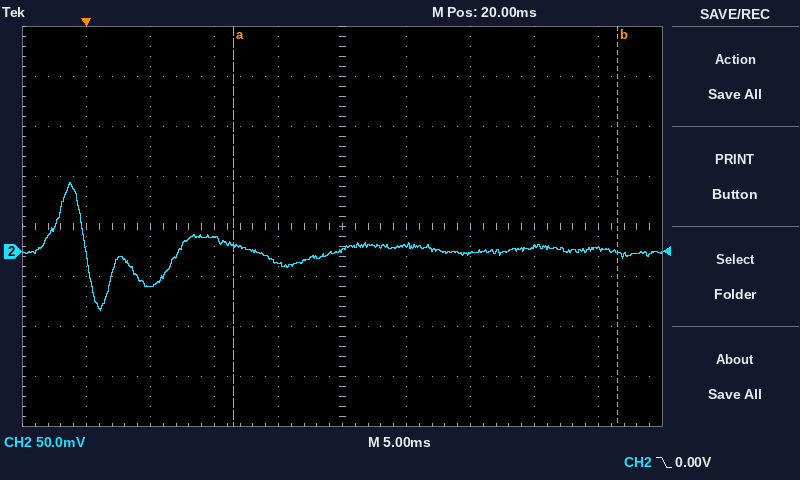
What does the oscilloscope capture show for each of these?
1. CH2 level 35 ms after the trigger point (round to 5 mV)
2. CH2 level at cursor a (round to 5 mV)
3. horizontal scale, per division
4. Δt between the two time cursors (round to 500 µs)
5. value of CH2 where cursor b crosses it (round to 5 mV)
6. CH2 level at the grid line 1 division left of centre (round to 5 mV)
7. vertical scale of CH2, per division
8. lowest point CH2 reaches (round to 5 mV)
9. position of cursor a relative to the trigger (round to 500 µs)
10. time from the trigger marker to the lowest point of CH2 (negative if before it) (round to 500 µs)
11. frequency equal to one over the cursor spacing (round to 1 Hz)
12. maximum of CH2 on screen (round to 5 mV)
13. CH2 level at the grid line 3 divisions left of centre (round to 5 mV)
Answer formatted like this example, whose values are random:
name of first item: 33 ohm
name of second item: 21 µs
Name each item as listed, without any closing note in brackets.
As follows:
CH2 level 35 ms after the trigger point: 5 mV
CH2 level at cursor a: 5 mV
horizontal scale, per division: 5 ms
Δt between the two time cursors: 30.0 ms
value of CH2 where cursor b crosses it: 0 mV
CH2 level at the grid line 1 division left of centre: -10 mV
vertical scale of CH2, per division: 50 mV
lowest point CH2 reaches: -60 mV
position of cursor a relative to the trigger: +11.5 ms
time from the trigger marker to the lowest point of CH2 (negative if before it): +1.0 ms
frequency equal to one over the cursor spacing: 33 Hz
maximum of CH2 on screen: 70 mV
CH2 level at the grid line 3 divisions left of centre: -35 mV
